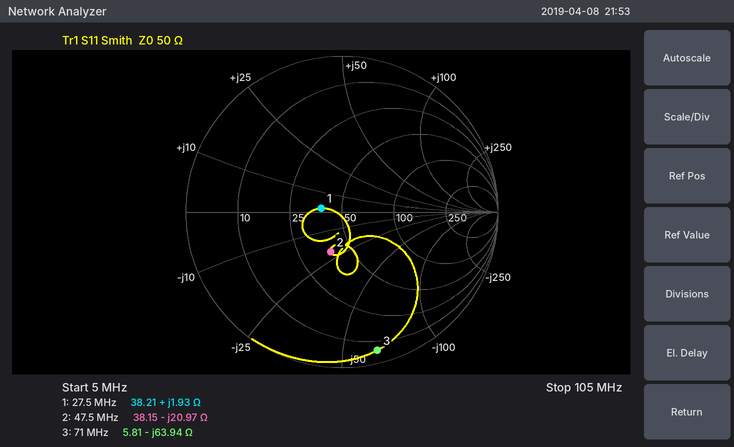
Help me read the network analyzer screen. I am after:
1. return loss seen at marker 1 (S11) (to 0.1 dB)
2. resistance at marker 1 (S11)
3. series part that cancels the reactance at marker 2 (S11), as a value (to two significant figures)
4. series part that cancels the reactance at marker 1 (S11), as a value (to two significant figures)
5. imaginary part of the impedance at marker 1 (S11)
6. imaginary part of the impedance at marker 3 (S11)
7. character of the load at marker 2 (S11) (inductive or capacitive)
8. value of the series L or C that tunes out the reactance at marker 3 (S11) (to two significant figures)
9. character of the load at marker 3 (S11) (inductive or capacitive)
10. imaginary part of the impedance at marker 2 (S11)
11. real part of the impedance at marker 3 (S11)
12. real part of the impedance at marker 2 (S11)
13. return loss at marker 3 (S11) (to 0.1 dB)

17.4 dB
38.21 Ω
70 nH
3.0 nF
+1.93 Ω
-63.94 Ω
capacitive
140 nH
capacitive
-20.97 Ω
5.81 Ω
38.15 Ω
0.8 dB
